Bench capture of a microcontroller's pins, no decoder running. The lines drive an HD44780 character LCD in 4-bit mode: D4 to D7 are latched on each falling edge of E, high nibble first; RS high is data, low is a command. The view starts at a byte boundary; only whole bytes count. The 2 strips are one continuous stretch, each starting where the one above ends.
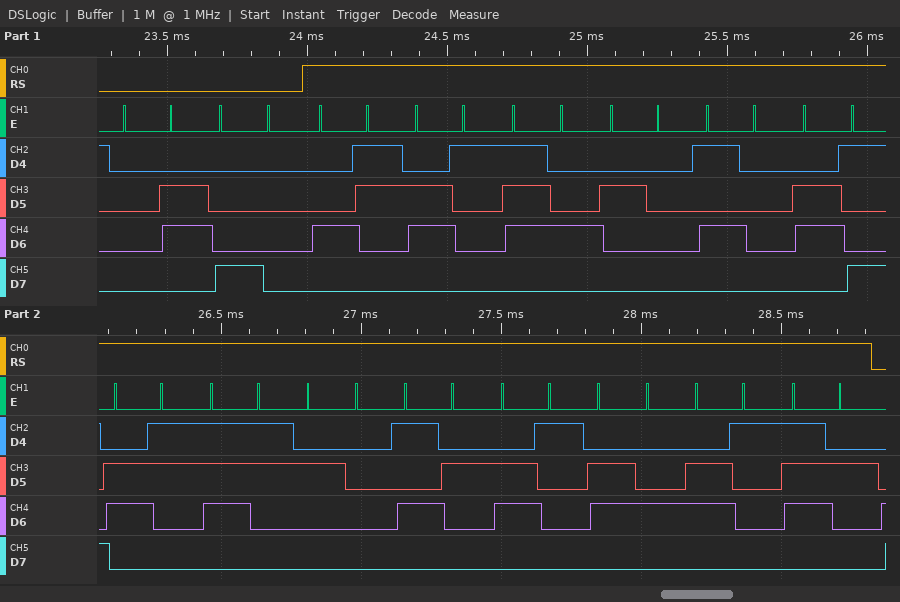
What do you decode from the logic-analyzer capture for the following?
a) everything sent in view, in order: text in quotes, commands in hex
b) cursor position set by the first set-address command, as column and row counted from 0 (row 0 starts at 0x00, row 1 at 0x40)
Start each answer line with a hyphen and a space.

- 0x06 0x80 "Cat Pics Radar"
- column 0, row 0
